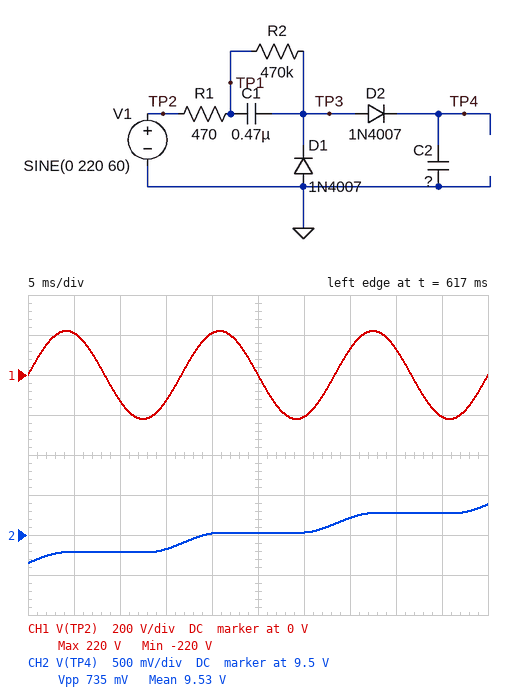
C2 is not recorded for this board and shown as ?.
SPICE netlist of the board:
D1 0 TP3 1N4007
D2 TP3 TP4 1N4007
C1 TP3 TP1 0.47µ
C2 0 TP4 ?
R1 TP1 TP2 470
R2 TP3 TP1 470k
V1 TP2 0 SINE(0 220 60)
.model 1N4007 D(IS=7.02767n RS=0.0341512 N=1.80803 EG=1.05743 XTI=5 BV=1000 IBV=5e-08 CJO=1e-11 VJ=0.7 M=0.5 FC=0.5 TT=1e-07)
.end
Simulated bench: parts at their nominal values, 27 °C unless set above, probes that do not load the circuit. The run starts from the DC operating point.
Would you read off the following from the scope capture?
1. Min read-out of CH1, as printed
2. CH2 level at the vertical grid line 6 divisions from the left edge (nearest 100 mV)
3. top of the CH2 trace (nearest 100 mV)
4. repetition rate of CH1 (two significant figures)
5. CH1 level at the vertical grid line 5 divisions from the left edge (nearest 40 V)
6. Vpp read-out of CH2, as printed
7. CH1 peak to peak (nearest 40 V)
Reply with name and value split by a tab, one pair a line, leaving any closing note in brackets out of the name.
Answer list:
Min read-out of CH1, as printed	-220 V
CH2 level at the vertical grid line 6 divisions from the left edge	9.5 V
top of the CH2 trace	9.9 V
repetition rate of CH1	60 Hz
CH1 level at the vertical grid line 5 divisions from the left edge	0 V
Vpp read-out of CH2, as printed	735 mV
CH1 peak to peak	440 V
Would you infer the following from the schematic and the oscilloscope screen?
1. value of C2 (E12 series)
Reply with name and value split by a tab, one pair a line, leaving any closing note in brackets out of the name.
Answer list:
value of C2	820 µF
